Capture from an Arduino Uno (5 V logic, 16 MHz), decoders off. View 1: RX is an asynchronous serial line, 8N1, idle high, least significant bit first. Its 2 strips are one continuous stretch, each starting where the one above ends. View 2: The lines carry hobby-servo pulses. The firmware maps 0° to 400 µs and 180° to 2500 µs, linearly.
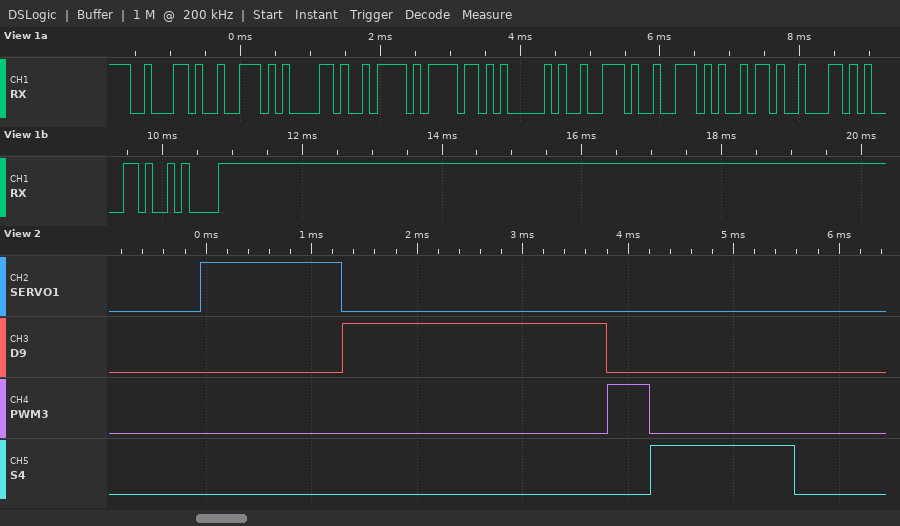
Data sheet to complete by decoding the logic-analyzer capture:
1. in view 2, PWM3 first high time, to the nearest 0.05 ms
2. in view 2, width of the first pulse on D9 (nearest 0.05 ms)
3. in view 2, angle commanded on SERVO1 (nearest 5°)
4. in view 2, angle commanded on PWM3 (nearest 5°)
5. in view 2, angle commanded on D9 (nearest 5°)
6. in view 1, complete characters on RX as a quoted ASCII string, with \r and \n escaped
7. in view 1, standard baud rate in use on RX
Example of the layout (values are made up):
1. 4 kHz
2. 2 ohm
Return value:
1. 0.40 ms
2. 2.50 ms
3. 80°
4. 0°
5. 180°
6. "brazoArriba\n"
7. 9600 baud
